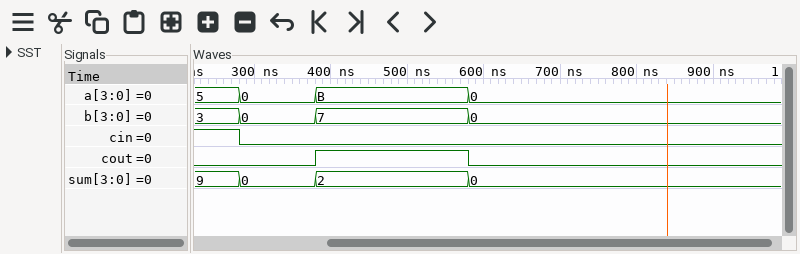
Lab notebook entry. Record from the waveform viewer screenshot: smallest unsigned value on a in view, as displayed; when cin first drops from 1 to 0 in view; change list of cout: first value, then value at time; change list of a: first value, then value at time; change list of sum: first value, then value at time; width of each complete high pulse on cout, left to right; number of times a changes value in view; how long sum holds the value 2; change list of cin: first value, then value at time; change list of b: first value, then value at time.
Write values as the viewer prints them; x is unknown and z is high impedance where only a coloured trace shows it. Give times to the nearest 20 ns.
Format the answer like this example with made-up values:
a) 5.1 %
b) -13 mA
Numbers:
a) 0
b) 280 ns
c) 0, 1 at 380 ns, 0 at 580 ns
d) 5, 0 at 280 ns, B at 380 ns, 0 at 580 ns
e) 9, 0 at 280 ns, 2 at 380 ns, 0 at 580 ns
f) 200 ns
g) 3
h) 200 ns
i) 1, 0 at 280 ns
j) 3, 0 at 280 ns, 7 at 380 ns, 0 at 580 ns
